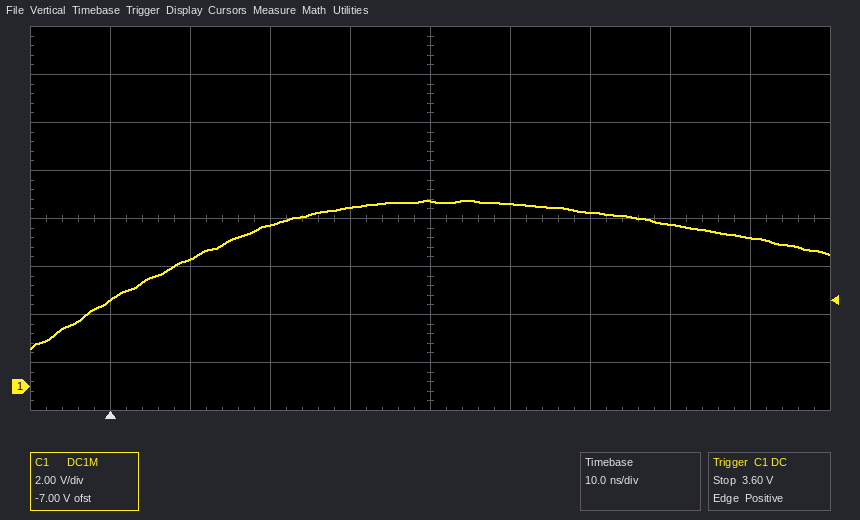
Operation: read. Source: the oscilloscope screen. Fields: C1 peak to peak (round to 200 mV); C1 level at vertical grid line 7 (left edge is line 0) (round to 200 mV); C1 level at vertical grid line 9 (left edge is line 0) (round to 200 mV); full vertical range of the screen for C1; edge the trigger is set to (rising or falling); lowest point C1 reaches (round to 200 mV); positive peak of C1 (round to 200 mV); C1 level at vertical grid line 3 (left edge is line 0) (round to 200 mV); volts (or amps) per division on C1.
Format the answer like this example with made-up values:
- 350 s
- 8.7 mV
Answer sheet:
- 6.2 V
- 7.2 V
- 6.2 V
- 16 V
- rising
- 1.6 V
- 7.8 V
- 6.8 V
- 2 V
